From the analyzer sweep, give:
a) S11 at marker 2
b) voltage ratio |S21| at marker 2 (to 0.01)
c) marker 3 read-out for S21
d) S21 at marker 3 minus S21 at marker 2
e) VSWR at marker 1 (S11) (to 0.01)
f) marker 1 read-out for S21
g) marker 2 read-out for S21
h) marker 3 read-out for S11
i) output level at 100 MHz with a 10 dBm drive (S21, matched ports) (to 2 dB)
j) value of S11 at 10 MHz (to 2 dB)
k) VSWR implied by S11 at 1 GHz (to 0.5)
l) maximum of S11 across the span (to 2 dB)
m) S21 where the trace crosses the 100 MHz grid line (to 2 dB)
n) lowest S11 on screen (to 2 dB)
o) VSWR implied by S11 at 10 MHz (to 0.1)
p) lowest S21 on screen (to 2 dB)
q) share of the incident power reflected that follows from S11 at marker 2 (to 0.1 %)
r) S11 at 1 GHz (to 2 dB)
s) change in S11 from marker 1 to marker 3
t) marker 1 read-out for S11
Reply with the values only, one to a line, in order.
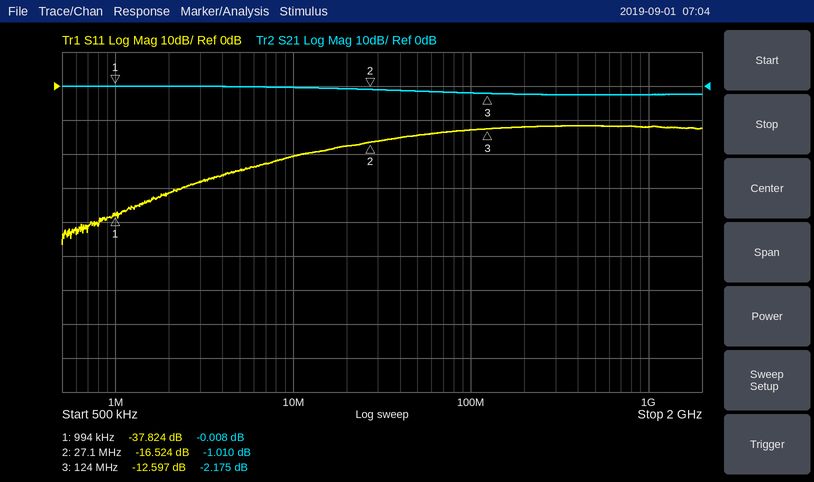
-16.524 dB
0.89
-2.175 dB
-1.165 dB
1.03
-0.008 dB
-1.010 dB
-12.597 dB
8 dBm
-20 dB
1.5
-12 dB
-2 dB
-46 dB
1.2
-2 dB
2.2 %
-12 dB
25.227 dB
-37.824 dB
